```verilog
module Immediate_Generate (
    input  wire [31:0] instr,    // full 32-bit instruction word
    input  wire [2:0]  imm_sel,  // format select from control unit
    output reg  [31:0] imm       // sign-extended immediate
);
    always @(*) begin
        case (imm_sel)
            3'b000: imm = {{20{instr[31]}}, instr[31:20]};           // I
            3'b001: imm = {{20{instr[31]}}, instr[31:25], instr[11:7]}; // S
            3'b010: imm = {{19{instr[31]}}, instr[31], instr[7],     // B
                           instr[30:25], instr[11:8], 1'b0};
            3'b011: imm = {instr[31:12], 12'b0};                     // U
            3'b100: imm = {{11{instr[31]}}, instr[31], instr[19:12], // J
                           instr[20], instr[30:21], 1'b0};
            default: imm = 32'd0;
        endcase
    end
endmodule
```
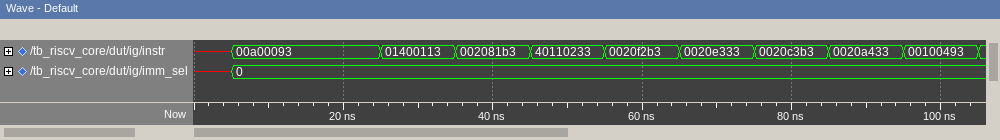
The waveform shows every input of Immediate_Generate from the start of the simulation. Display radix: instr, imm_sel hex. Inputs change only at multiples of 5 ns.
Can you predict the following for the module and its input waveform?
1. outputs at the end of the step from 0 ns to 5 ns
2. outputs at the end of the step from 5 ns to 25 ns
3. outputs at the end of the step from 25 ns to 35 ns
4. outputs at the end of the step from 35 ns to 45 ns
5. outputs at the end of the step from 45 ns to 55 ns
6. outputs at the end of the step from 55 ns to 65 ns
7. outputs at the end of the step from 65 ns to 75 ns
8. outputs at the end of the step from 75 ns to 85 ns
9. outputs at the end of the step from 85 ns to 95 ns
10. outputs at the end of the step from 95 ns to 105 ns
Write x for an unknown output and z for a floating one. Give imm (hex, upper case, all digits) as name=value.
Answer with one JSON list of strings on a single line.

["imm=x", "imm=0000000A", "imm=00000014", "imm=00000002", "imm=00000401", "imm=00000002", "imm=00000002", "imm=00000002", "imm=00000002", "imm=00000001"]
